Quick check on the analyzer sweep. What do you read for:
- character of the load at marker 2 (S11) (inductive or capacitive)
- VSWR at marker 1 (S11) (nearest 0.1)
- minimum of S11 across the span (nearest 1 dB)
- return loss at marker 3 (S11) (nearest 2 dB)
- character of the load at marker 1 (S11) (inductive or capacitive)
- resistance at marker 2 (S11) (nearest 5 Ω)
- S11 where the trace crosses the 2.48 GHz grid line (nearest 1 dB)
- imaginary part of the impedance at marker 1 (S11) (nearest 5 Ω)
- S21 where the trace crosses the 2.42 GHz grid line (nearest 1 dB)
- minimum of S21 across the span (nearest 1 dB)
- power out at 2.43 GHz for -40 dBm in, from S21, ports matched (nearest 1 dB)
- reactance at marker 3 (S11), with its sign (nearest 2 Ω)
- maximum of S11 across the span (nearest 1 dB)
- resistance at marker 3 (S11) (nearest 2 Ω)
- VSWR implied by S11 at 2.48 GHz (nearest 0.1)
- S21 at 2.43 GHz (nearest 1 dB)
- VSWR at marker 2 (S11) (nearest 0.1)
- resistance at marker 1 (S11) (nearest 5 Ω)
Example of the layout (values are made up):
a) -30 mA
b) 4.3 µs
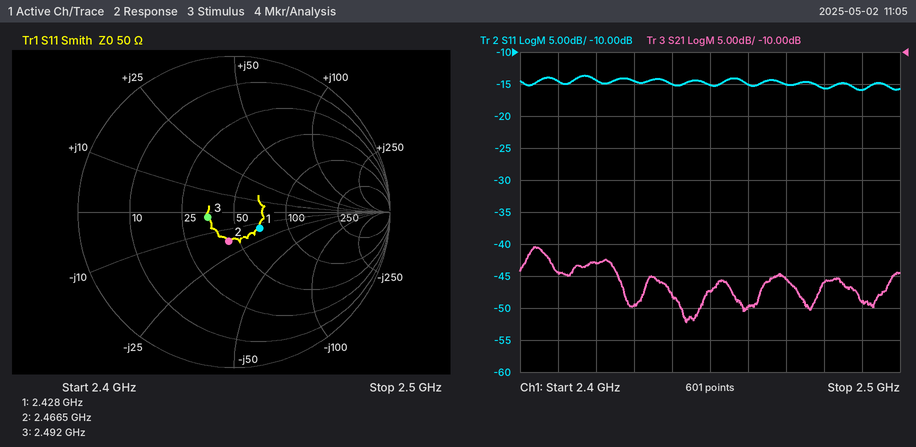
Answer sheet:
a) capacitive
b) 1.5
c) -16 dB
d) 16 dB
e) capacitive
f) 45 Ω
g) -16 dB
h) -15 Ω
i) -43 dB
j) -52 dB
k) -90 dBm
l) -2 Ω
m) -14 dB
n) 36 Ω
o) 1.4
p) -50 dB
q) 1.5
r) 70 Ω
